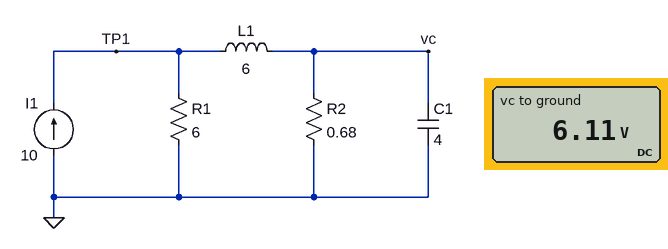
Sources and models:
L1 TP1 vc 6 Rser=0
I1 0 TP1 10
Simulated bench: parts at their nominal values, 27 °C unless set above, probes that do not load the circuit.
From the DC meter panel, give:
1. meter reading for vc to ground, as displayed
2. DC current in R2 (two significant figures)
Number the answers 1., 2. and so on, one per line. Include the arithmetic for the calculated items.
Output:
1. 6.11 V
2. (6.11 V) / 680 mΩ = 9.0 A
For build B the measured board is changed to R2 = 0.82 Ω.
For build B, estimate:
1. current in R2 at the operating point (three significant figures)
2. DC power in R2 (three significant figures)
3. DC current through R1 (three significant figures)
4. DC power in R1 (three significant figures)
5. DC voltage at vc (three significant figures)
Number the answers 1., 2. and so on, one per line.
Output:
1. 8.80 A
2. 63.5 W
3. 1.20 A
4. 8.67 W
5. 7.21 V
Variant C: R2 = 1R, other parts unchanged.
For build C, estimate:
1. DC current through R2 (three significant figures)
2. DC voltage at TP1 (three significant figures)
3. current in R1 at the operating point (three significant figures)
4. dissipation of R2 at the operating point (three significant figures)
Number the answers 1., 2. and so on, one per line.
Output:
1. 8.57 A
2. 8.57 V
3. 1.43 A
4. 73.5 W
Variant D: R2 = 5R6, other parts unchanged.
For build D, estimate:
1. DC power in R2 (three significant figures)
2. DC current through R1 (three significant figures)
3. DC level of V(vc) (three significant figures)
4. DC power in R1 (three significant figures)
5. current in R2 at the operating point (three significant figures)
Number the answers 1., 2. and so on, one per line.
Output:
1. 150 W
2. 4.83 A
3. 29.0 V
4. 140 W
5. 5.17 A
